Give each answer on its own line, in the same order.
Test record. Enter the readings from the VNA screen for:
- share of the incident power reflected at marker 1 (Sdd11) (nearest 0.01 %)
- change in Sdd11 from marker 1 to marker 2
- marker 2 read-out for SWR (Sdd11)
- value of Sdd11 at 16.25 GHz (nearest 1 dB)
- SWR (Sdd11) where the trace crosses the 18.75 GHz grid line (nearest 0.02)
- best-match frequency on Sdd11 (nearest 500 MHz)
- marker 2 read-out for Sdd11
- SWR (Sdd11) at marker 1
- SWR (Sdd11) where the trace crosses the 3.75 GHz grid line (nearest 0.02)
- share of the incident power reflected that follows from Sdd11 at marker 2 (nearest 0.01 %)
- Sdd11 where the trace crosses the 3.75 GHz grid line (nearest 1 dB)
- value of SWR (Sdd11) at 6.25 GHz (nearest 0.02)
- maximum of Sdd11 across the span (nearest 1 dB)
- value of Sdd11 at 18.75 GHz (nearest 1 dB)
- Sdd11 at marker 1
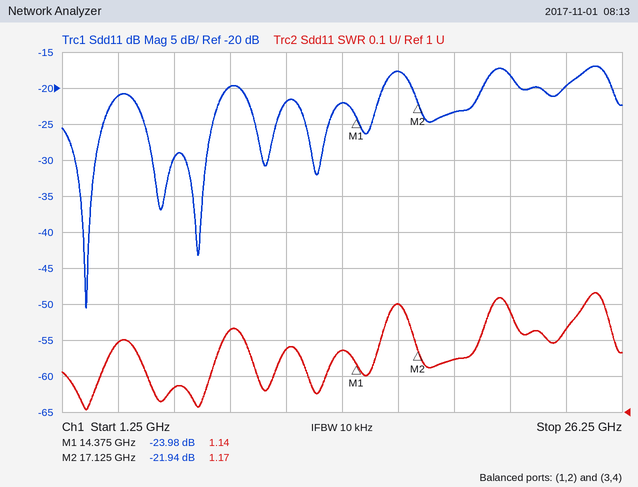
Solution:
0.40 %
2.04 dB
1.17
-18 dB
1.14
2.5 GHz
-21.94 dB
1.14
1.20
0.64 %
-21 dB
1.06
-17 dB
-23 dB
-23.98 dB
